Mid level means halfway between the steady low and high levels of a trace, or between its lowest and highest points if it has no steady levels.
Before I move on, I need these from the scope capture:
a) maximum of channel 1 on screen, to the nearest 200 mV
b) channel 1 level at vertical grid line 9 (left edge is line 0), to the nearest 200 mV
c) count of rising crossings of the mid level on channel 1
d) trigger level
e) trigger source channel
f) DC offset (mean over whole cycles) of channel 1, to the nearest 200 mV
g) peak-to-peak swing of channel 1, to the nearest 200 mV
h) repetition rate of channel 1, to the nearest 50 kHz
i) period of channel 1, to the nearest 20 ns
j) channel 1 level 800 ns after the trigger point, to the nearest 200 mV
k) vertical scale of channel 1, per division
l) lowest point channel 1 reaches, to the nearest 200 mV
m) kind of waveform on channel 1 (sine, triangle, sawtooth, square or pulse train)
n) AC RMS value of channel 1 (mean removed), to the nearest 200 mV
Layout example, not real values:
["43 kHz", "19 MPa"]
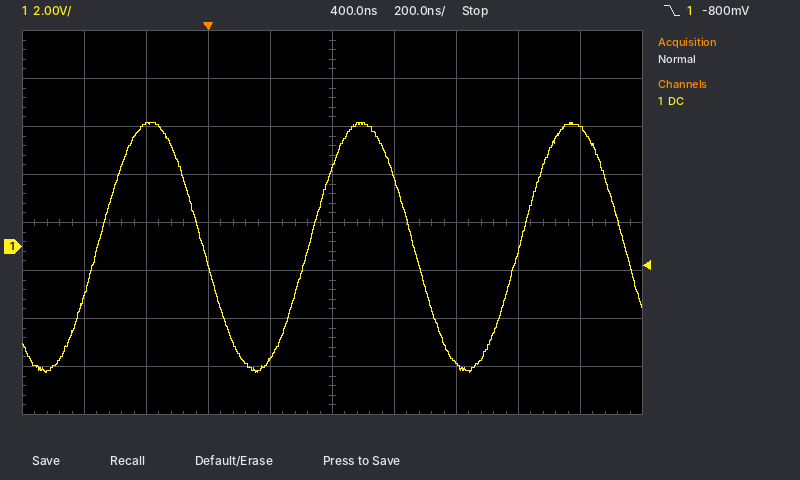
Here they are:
["5.2 V", "5.0 V", "3", "-800 mV", "channel 1", "0.0 V", "10.4 V", "1.45 MHz", "680 ns", "-4.8 V", "2 V", "-5.2 V", "sine", "3.6 V"]
